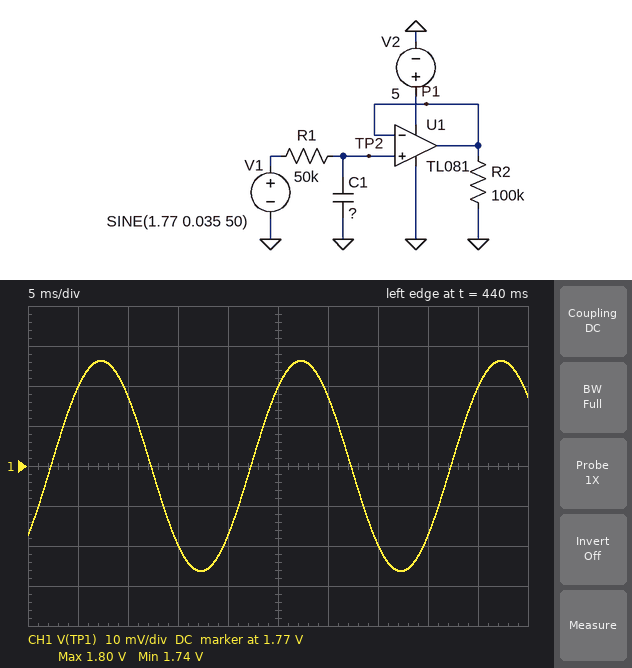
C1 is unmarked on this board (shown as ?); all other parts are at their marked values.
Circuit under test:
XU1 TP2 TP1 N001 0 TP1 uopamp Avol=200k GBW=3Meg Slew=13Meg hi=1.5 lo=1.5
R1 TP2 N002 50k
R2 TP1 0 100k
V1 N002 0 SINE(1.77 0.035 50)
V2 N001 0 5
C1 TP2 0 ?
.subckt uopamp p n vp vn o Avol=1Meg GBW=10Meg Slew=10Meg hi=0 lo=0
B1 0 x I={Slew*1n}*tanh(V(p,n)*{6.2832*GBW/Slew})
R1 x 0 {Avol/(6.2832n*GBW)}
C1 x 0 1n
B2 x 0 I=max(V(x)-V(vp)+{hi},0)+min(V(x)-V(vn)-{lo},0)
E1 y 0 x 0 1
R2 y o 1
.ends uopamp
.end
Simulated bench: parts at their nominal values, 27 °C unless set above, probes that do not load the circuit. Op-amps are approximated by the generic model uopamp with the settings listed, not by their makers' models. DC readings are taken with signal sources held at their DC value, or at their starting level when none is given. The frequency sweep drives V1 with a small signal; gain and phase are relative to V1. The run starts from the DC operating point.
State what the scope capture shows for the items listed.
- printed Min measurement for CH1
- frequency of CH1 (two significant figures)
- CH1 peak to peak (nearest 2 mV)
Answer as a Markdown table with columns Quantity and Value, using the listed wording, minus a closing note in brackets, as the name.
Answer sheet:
| Quantity | Value |
|---|---|
| printed Min measurement for CH1 | 1.74 V |
| frequency of CH1 | 50 Hz |
| CH1 peak to peak | 52 mV |
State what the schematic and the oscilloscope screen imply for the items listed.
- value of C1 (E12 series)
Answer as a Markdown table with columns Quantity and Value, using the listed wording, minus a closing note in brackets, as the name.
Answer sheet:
| Quantity | Value |
|---|---|
| value of C1 | 56 nF |
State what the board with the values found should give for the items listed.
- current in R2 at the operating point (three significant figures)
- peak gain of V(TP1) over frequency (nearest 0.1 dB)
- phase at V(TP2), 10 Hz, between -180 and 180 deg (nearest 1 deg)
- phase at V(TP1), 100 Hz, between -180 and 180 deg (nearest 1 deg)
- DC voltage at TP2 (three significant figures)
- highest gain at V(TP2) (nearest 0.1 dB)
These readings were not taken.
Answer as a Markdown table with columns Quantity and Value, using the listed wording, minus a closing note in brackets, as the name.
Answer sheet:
| Quantity | Value |
|---|---|
| current in R2 at the operating point | 17.7 µA |
| peak gain of V(TP1) over frequency | 0 dB |
| phase at V(TP2), 10 Hz, between -180 and 180 deg | -10 deg |
| phase at V(TP1), 100 Hz, between -180 and 180 deg | -60 deg |
| DC voltage at TP2 | 1.77 V |
| highest gain at V(TP2) | 0 dB |
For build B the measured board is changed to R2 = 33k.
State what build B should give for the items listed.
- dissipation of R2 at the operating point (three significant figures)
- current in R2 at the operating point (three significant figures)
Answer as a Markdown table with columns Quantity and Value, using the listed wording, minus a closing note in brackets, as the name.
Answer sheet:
| Quantity | Value |
|---|---|
| dissipation of R2 at the operating point | 94.9 µW |
| current in R2 at the operating point | 53.6 µA |
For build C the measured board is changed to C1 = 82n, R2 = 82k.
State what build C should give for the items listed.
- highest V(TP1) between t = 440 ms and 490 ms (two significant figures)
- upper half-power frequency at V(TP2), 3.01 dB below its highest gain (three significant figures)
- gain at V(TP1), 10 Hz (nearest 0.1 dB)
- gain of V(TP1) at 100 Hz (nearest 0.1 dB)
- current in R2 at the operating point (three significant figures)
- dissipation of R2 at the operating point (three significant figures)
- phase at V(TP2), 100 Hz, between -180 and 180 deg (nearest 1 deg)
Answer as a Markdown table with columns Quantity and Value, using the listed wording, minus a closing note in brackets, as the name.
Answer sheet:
| Quantity | Value |
|---|---|
| highest V(TP1) between t = 440 ms and 490 ms | 1.8 V |
| upper half-power frequency at V(TP2), 3.01 dB below its highest gain | 38.8 Hz |
| gain at V(TP1), 10 Hz | -0.3 dB |
| gain of V(TP1) at 100 Hz | -8.8 dB |
| current in R2 at the operating point | 21.6 µA |
| dissipation of R2 at the operating point | 38.2 µW |
| phase at V(TP2), 100 Hz, between -180 and 180 deg | -69 deg |
